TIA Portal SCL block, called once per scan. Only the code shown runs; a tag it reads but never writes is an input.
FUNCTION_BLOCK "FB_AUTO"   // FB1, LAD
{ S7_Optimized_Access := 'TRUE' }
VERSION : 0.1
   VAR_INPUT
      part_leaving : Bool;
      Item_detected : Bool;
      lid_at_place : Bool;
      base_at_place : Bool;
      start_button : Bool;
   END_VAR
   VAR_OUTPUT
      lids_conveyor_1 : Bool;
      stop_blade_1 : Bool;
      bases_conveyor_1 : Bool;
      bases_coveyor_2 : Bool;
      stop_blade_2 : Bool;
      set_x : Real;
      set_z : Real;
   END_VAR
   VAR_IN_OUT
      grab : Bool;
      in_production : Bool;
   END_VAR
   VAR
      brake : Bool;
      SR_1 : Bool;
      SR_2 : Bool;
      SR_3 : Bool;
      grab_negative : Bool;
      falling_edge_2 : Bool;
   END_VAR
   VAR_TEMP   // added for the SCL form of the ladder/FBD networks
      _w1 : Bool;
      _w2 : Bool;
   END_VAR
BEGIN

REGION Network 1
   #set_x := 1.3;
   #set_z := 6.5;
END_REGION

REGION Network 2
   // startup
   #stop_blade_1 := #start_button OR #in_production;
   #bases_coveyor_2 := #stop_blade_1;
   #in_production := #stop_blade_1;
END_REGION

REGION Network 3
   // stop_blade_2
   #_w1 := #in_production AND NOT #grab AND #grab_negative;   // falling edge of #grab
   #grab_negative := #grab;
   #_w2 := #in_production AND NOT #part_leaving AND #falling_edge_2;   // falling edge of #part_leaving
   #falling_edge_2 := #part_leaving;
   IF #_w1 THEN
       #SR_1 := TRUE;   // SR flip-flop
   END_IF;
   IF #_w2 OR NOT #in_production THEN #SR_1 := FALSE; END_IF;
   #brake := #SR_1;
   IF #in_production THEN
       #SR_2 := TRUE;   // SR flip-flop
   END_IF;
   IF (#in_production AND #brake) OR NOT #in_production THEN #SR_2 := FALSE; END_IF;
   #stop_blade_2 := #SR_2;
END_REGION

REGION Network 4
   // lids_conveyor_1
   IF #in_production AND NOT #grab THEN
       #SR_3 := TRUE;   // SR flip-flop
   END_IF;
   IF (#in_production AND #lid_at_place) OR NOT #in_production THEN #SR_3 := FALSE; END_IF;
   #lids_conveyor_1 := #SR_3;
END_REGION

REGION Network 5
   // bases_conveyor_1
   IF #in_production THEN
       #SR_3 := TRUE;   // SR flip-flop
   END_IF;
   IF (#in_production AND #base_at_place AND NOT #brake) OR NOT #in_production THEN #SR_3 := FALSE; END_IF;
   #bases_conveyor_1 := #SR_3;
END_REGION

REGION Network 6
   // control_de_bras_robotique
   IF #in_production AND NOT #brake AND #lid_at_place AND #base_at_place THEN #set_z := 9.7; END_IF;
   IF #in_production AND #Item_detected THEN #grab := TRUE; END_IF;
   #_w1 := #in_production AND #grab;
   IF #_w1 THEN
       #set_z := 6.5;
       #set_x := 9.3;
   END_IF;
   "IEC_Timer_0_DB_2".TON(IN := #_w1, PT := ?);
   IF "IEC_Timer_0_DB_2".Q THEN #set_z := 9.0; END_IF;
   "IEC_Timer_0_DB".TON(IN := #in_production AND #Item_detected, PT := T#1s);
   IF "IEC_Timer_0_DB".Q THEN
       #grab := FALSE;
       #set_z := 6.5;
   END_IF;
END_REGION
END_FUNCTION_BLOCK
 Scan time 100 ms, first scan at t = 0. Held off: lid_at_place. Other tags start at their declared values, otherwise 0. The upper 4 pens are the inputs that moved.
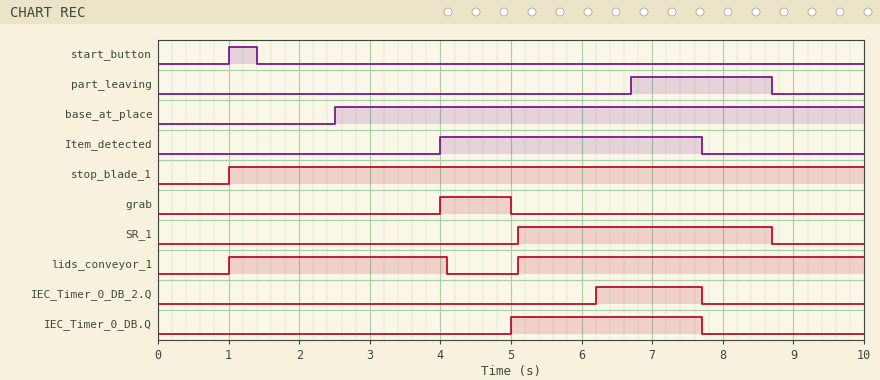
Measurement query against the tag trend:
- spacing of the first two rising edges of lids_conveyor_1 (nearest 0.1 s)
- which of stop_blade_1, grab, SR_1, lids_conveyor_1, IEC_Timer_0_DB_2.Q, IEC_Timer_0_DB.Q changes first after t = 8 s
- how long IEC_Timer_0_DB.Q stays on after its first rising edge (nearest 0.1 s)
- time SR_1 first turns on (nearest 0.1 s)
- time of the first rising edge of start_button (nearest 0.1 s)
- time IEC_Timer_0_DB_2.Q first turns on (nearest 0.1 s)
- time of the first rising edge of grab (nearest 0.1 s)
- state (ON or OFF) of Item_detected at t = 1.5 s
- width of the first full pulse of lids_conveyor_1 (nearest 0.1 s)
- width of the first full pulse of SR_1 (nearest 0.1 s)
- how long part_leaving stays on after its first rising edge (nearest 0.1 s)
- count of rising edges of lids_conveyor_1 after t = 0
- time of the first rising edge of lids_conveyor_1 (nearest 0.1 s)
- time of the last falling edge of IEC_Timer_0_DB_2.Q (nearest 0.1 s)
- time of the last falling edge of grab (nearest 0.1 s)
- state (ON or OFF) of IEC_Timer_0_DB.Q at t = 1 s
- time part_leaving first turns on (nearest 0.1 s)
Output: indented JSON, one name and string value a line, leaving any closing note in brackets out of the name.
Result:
{
  "spacing of the first two rising edges of lids_conveyor_1": "4.1 s",
  "which of stop_blade_1, grab, SR_1, lids_conveyor_1, IEC_Timer_0_DB_2.Q, IEC_Timer_0_DB.Q changes first after t = 8 s": "SR_1",
  "how long IEC_Timer_0_DB.Q stays on after its first rising edge": "2.7 s",
  "time SR_1 first turns on": "5.1 s",
  "time of the first rising edge of start_button": "1.0 s",
  "time IEC_Timer_0_DB_2.Q first turns on": "6.2 s",
  "time of the first rising edge of grab": "4.0 s",
  "state (ON or OFF) of Item_detected at t = 1.5 s": "OFF",
  "width of the first full pulse of lids_conveyor_1": "3.1 s",
  "width of the first full pulse of SR_1": "3.6 s",
  "how long part_leaving stays on after its first rising edge": "2.0 s",
  "count of rising edges of lids_conveyor_1 after t = 0": "2",
  "time of the first rising edge of lids_conveyor_1": "1.0 s",
  "time of the last falling edge of IEC_Timer_0_DB_2.Q": "7.7 s",
  "time of the last falling edge of grab": "5.0 s",
  "state (ON or OFF) of IEC_Timer_0_DB.Q at t = 1 s": "OFF",
  "time part_leaving first turns on": "6.7 s"
}
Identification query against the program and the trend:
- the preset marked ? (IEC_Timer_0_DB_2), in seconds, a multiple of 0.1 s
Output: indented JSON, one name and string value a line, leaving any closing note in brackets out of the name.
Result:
{
  "the preset marked ? (IEC_Timer_0_DB_2), in seconds, a multiple of 0.1 s": "2.2 s"
}
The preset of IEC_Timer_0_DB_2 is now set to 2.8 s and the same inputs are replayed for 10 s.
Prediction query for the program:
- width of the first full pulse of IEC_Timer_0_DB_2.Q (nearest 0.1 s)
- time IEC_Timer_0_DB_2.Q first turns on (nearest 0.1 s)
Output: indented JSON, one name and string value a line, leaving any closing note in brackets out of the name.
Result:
{
  "width of the first full pulse of IEC_Timer_0_DB_2.Q": "0.9 s",
  "time IEC_Timer_0_DB_2.Q first turns on": "6.8 s"
}
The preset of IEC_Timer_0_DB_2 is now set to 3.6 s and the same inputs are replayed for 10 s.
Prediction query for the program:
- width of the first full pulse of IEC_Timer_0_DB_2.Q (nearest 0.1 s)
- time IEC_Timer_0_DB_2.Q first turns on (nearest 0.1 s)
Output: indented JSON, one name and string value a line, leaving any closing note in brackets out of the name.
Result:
{
  "width of the first full pulse of IEC_Timer_0_DB_2.Q": "0.1 s",
  "time IEC_Timer_0_DB_2.Q first turns on": "7.6 s"
}
